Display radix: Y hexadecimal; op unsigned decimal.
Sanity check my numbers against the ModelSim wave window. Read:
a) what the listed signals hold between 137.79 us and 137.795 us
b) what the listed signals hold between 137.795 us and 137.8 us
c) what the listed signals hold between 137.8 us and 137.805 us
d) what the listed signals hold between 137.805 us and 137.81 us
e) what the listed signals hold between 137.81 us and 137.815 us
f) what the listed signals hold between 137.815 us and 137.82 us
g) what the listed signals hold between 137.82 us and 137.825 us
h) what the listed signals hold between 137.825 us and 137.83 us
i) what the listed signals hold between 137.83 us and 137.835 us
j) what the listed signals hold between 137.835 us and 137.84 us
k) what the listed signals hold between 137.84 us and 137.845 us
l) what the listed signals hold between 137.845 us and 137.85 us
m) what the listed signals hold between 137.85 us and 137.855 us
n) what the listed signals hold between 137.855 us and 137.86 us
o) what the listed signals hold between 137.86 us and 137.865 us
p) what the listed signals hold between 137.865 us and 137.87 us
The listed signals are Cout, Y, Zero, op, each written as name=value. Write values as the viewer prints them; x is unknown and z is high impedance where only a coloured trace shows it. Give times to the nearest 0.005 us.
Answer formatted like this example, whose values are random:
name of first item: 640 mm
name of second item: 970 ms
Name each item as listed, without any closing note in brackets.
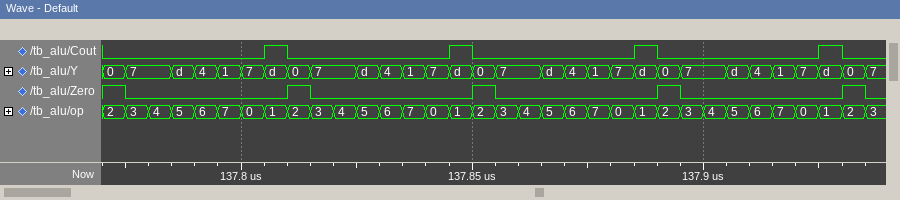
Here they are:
what the listed signals hold between 137.79 us and 137.795 us: Cout=0, Y=4, Zero=0, op=6
what the listed signals hold between 137.795 us and 137.8 us: Cout=0, Y=1, Zero=0, op=7
what the listed signals hold between 137.8 us and 137.805 us: Cout=0, Y=7, Zero=0, op=0
what the listed signals hold between 137.805 us and 137.81 us: Cout=1, Y=d, Zero=0, op=1
what the listed signals hold between 137.81 us and 137.815 us: Cout=0, Y=0, Zero=1, op=2
what the listed signals hold between 137.815 us and 137.82 us: Cout=0, Y=7, Zero=0, op=3
what the listed signals hold between 137.82 us and 137.825 us: Cout=0, Y=7, Zero=0, op=4
what the listed signals hold between 137.825 us and 137.83 us: Cout=0, Y=d, Zero=0, op=5
what the listed signals hold between 137.83 us and 137.835 us: Cout=0, Y=4, Zero=0, op=6
what the listed signals hold between 137.835 us and 137.84 us: Cout=0, Y=1, Zero=0, op=7
what the listed signals hold between 137.84 us and 137.845 us: Cout=0, Y=7, Zero=0, op=0
what the listed signals hold between 137.845 us and 137.85 us: Cout=1, Y=d, Zero=0, op=1
what the listed signals hold between 137.85 us and 137.855 us: Cout=0, Y=0, Zero=1, op=2
what the listed signals hold between 137.855 us and 137.86 us: Cout=0, Y=7, Zero=0, op=3
what the listed signals hold between 137.86 us and 137.865 us: Cout=0, Y=7, Zero=0, op=4
what the listed signals hold between 137.865 us and 137.87 us: Cout=0, Y=d, Zero=0, op=5
